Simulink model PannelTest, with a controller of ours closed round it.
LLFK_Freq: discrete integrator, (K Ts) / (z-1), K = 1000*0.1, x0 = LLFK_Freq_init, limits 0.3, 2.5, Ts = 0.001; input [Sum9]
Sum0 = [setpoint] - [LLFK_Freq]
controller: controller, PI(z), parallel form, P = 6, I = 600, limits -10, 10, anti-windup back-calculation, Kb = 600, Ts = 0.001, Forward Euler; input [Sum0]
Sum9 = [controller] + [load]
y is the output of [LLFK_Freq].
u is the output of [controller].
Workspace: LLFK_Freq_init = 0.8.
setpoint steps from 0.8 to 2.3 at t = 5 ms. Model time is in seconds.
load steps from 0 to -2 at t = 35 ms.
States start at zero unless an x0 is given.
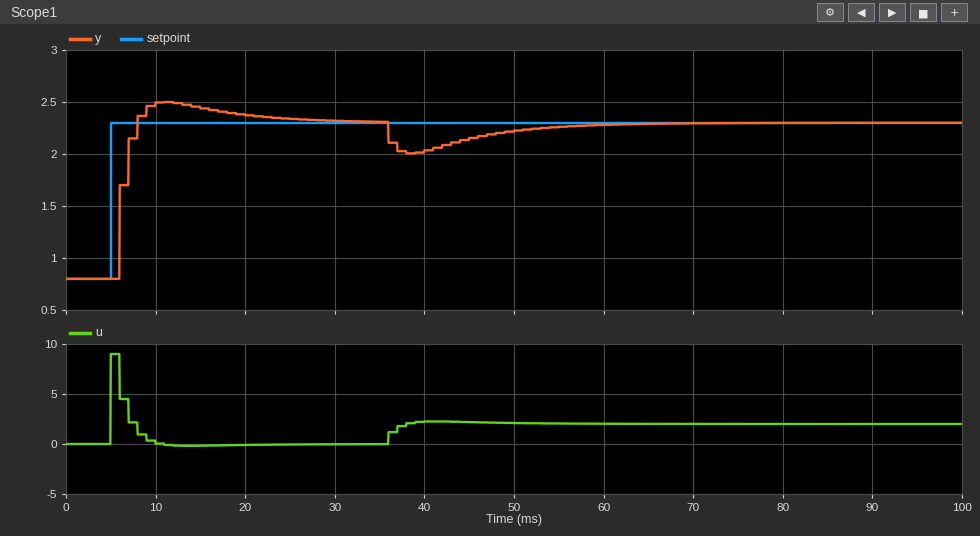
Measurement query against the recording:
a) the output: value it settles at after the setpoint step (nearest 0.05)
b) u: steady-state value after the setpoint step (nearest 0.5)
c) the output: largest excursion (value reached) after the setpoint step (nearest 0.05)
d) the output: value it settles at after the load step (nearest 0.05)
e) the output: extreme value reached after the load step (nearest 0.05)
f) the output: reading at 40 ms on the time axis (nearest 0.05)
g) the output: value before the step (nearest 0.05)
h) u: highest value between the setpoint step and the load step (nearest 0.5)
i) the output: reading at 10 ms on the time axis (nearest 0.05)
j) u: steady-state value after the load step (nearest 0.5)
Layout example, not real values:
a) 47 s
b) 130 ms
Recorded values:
a) 2.30
b) 0.0
c) 2.50
d) 2.30
e) 2.00
f) 2.05
g) 0.80
h) 9.0
i) 2.50
j) 2.0
